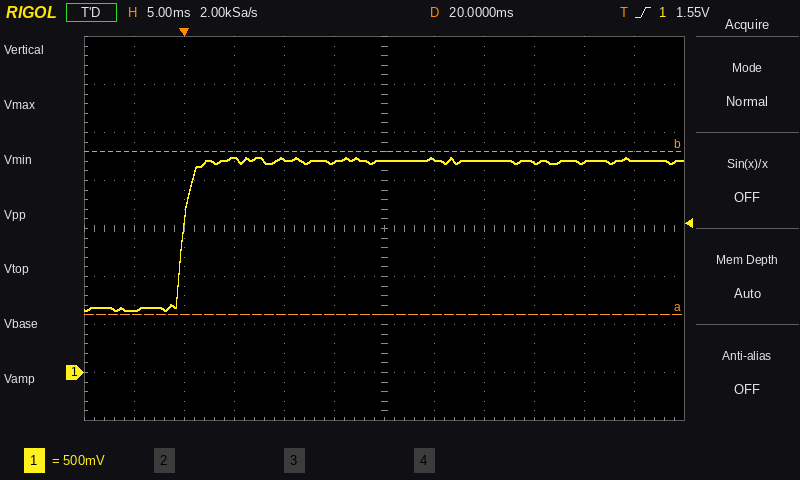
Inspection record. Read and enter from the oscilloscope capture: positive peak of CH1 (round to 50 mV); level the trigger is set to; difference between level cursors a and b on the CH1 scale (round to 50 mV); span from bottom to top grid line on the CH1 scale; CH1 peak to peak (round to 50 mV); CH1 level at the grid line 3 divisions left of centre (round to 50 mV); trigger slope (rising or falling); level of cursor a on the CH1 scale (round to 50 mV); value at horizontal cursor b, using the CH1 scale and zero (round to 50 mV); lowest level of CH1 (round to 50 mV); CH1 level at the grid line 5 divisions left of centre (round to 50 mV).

2.25 V
1.55 V
1.70 V
4 V
1.60 V
2.25 V
rising
600 mV
2.30 V
650 mV
650 mV
